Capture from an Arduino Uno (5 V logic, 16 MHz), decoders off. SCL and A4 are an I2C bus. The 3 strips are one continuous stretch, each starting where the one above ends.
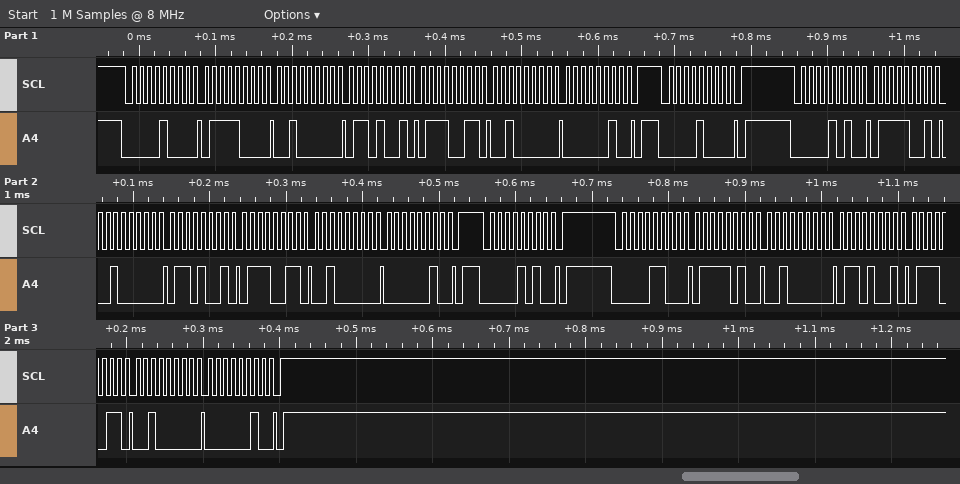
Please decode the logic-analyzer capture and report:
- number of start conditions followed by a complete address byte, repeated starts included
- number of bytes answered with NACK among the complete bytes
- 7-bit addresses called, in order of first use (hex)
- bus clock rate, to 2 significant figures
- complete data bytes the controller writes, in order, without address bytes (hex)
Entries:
5
0
0x04 0x05 0x06
100 kHz
78 20 69 73 20 02 79 20 69 73 20 02 7A 20 69 73 20 02
